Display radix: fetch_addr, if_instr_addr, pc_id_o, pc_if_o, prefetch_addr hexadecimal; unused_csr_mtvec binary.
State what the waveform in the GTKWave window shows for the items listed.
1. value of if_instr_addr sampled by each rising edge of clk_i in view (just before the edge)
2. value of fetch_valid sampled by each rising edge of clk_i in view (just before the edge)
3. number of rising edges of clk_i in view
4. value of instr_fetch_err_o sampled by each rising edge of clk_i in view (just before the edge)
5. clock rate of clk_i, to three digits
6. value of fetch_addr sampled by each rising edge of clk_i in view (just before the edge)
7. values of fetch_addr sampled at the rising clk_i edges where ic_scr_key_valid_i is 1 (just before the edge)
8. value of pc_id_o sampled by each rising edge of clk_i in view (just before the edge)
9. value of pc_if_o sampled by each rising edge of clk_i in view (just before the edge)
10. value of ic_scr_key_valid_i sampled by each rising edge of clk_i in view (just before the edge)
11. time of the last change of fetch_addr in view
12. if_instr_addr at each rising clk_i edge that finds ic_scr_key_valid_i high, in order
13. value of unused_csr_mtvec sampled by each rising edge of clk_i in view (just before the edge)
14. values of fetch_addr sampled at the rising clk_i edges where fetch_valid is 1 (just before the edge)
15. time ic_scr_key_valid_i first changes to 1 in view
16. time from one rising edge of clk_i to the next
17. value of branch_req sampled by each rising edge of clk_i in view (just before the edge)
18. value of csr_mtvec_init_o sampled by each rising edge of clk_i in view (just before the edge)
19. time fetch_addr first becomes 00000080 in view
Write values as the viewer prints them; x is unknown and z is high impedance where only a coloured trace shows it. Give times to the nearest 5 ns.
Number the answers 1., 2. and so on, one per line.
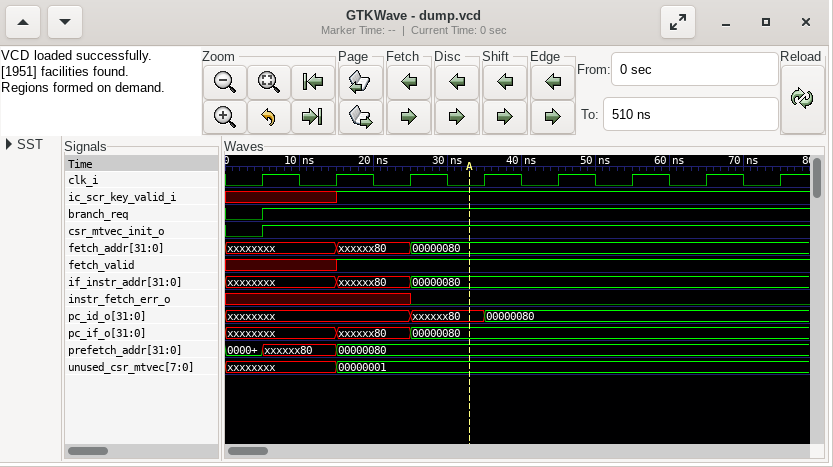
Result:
1. xxxxxxxx, xxxxxxxx, xxxxxx80, 00000080, 00000080, 00000080, 00000080, 00000080
2. x x 1 1 1 1 1 1
3. 8
4. x x x 0 0 0 0 0
5. 100 MHz
6. xxxxxxxx, xxxxxxxx, xxxxxx80, 00000080, 00000080, 00000080, 00000080, 00000080
7. xxxxxx80, 00000080, 00000080, 00000080, 00000080, 00000080
8. xxxxxxxx, xxxxxxxx, xxxxxxxx, xxxxxx80, 00000080, 00000080, 00000080, 00000080
9. xxxxxxxx, xxxxxxxx, xxxxxx80, 00000080, 00000080, 00000080, 00000080, 00000080
10. x x 1 1 1 1 1 1
11. 25 ns
12. xxxxxx80, 00000080, 00000080, 00000080, 00000080, 00000080
13. xxxxxxxx, xxxxxxxx, 00000001, 00000001, 00000001, 00000001, 00000001, 00000001
14. xxxxxx80, 00000080, 00000080, 00000080, 00000080, 00000080
15. 15 ns
16. 10 ns
17. 0 1 1 1 1 1 1 1
18. 0 1 1 1 1 1 1 1
19. 25 ns
